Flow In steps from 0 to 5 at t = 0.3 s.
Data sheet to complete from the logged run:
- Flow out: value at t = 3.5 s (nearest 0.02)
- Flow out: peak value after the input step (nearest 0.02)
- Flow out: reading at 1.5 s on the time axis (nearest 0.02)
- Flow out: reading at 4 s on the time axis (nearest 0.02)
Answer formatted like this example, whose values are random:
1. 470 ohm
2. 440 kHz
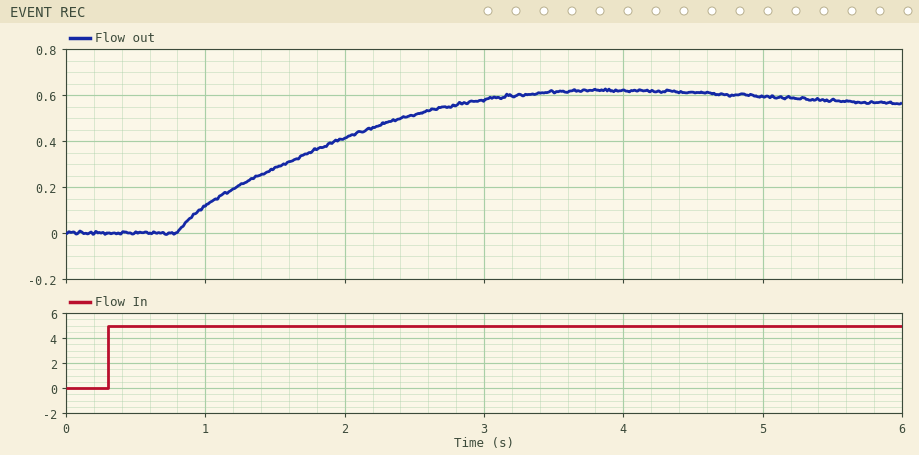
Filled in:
1. 0.62
2. 0.62
3. 0.28
4. 0.62
